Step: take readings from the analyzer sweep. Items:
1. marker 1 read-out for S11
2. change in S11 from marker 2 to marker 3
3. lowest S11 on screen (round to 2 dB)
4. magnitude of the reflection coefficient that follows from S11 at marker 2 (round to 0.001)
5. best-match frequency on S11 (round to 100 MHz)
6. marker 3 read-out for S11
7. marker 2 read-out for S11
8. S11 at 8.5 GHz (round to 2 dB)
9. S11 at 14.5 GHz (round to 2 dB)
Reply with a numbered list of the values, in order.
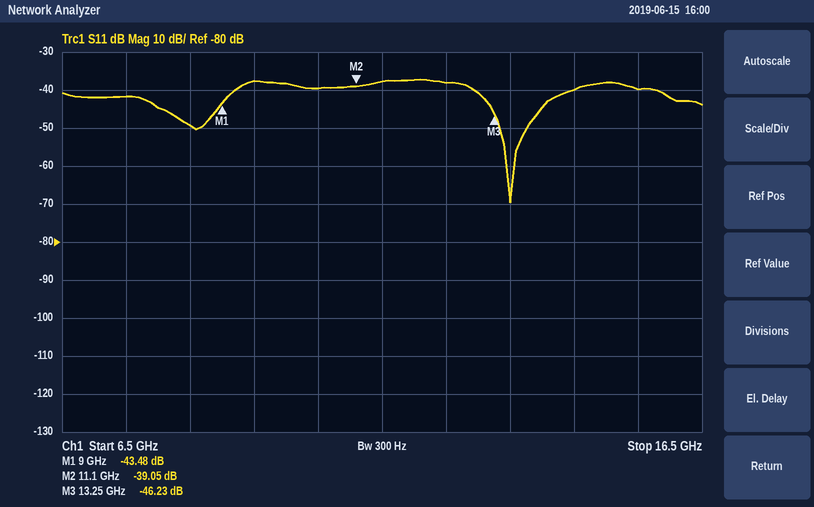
1. -43.48 dB
2. -7.18 dB
3. -70 dB
4. 0.011
5. 13.5 GHz
6. -46.23 dB
7. -39.05 dB
8. -50 dB
9. -40 dB
